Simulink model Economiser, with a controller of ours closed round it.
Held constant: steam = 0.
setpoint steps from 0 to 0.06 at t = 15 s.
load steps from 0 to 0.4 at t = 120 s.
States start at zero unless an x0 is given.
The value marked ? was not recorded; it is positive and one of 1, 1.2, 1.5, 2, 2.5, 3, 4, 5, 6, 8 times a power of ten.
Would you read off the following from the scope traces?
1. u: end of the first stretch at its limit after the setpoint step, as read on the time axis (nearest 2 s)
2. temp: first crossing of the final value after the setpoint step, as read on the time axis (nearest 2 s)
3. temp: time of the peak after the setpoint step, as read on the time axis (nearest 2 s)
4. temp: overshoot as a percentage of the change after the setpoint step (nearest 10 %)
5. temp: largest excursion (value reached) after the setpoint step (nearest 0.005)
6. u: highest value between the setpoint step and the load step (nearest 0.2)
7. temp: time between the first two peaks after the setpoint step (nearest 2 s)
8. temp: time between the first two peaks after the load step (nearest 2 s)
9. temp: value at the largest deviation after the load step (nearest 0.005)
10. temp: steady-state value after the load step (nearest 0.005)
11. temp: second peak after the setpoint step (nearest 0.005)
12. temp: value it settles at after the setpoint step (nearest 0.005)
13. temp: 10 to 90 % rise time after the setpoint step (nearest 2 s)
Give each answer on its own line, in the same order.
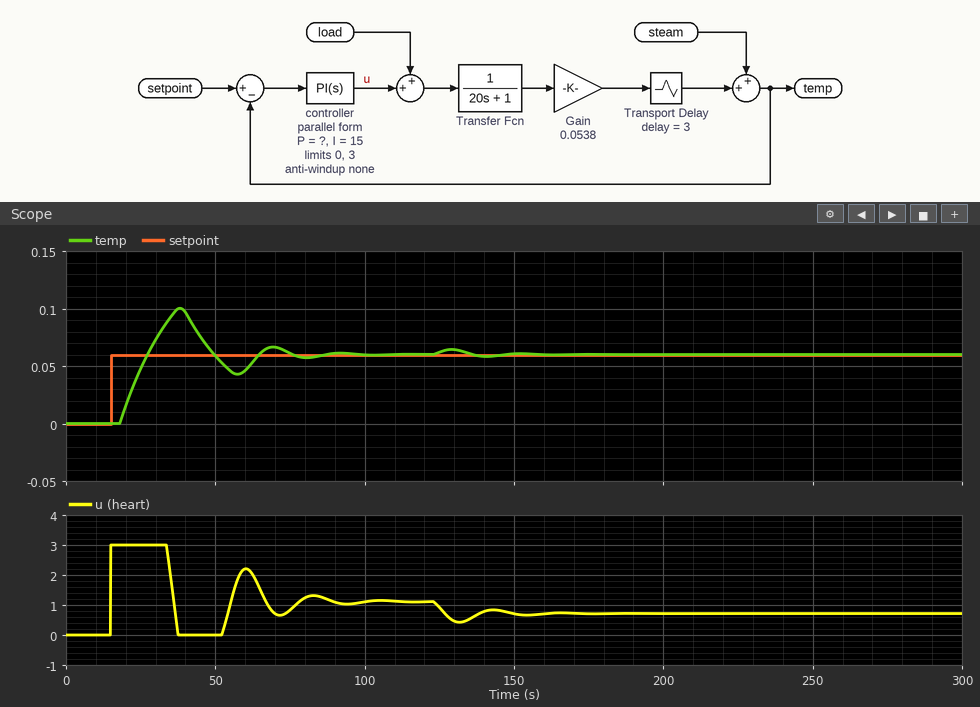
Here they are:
34 s
28 s
38 s
70 %
0.100
3.0
32 s
22 s
0.065
0.060
0.065
0.060
8 s
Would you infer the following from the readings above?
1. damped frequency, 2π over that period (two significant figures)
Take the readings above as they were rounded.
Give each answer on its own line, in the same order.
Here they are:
0.20 rad/s
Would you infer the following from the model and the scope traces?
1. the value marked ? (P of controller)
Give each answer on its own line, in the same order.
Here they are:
80
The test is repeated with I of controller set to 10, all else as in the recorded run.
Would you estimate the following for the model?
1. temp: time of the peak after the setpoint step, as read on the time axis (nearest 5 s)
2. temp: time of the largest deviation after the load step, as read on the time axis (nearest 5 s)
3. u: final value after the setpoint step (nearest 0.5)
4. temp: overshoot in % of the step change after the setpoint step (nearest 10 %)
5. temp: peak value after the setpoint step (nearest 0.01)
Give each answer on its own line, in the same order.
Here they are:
35 s
130 s
1.0
50 %
0.09
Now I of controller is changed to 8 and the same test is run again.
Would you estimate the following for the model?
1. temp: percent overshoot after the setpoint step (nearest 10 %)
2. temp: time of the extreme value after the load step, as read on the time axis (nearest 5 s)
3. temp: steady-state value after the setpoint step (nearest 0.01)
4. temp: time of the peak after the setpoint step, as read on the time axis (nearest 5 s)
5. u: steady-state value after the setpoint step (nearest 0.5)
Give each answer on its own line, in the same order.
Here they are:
40 %
130 s
0.06
35 s
1.0
